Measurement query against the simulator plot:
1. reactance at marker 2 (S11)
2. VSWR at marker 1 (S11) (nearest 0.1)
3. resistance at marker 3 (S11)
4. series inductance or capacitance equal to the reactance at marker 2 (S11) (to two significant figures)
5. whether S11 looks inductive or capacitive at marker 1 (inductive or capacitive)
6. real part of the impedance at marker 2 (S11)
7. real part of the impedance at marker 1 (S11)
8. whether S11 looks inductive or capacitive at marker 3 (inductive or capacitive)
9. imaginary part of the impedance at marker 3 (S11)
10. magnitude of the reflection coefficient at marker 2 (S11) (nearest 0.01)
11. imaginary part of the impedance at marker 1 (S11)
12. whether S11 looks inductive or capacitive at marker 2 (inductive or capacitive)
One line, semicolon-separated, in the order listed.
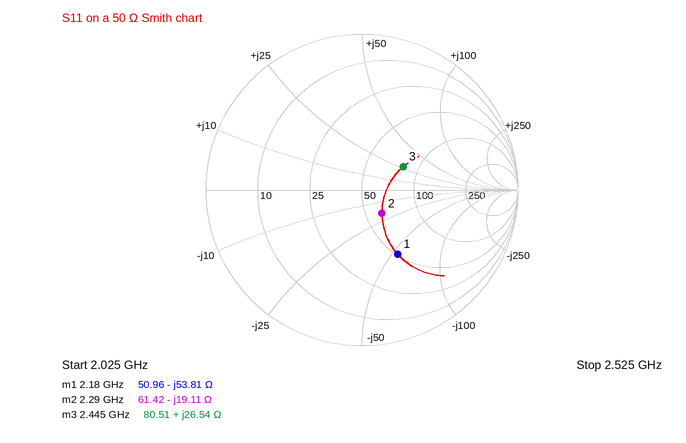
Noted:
-19.11 Ω; 2.8; 80.51 Ω; 3.6 pF; capacitive; 61.42 Ω; 50.96 Ω; inductive; +26.54 Ω; 0.20; -53.81 Ω; capacitive
